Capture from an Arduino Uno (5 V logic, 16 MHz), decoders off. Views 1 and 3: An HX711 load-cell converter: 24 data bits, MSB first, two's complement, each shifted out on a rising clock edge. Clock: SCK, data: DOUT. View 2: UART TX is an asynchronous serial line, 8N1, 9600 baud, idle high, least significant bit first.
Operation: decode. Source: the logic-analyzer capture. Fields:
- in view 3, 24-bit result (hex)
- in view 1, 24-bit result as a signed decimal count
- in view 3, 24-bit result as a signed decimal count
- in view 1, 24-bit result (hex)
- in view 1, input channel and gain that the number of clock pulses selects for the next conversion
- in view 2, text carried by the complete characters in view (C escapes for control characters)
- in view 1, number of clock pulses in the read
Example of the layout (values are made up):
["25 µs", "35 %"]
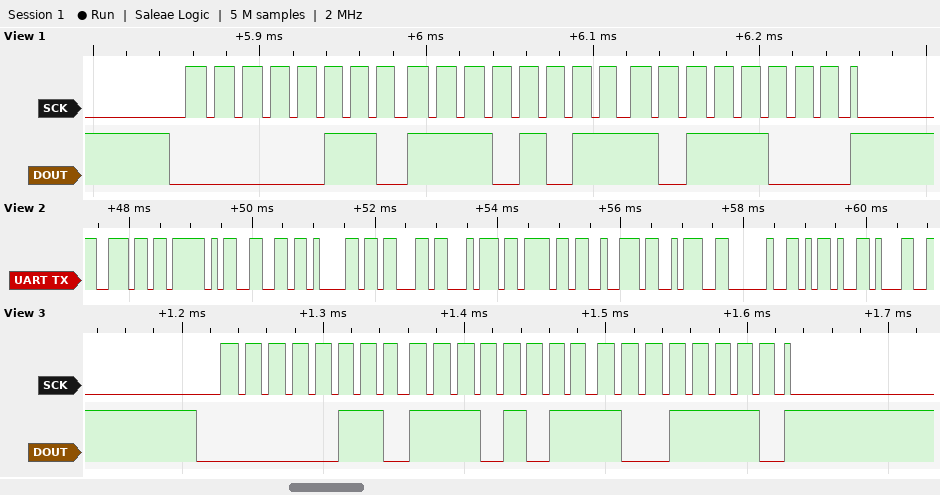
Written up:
["0x06EB9E", "453560", "453534", "0x06EBB8", "channel A, gain 128", "\"n_factor: -1\"", "25"]
